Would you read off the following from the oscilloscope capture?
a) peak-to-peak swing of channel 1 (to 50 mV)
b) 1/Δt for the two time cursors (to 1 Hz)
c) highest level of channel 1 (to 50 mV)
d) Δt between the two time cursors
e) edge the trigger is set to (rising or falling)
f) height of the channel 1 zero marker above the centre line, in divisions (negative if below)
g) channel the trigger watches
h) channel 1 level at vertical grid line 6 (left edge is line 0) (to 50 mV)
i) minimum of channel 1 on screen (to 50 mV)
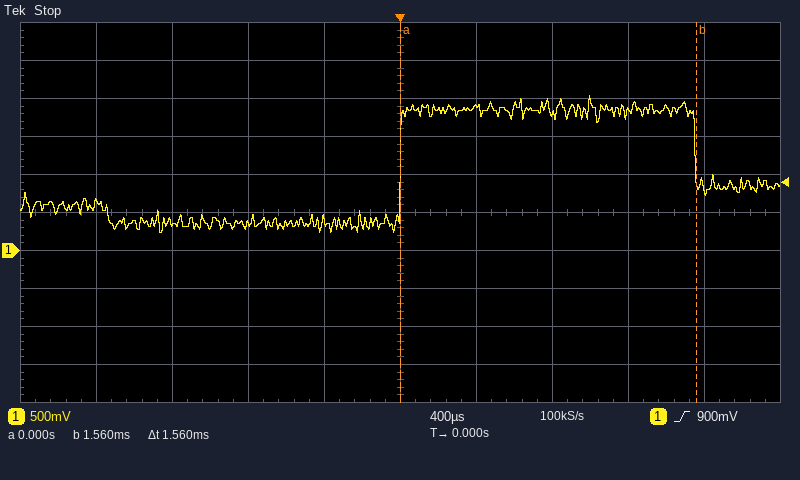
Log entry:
1.80 V
641 Hz
2.05 V
1.56 ms
rising
-1.0 div
channel 1
1.90 V
250 mV
